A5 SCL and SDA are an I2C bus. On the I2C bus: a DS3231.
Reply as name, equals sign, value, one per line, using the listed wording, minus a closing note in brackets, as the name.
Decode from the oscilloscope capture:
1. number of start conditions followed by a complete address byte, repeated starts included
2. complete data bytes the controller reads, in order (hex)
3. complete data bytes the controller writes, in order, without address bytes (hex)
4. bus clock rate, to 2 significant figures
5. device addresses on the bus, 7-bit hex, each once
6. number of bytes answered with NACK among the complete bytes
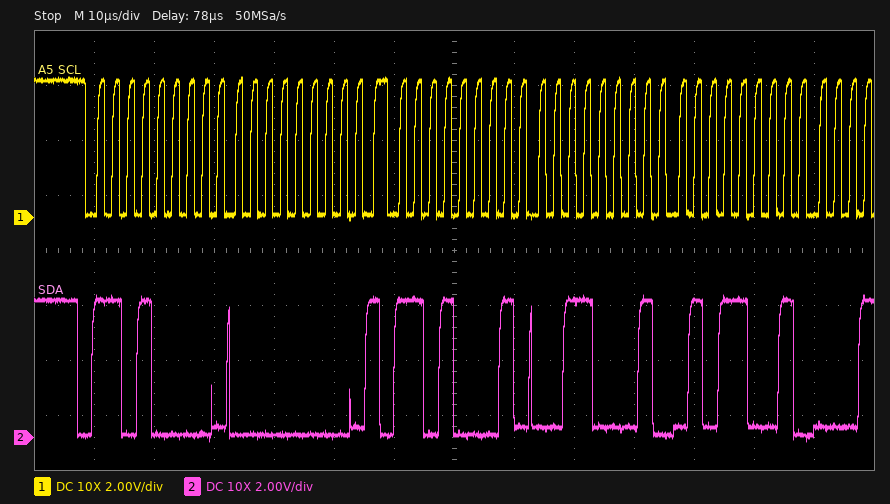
number of start conditions followed by a complete address byte, repeated starts included = 2
complete data bytes the controller reads, in order = 31 59
complete data bytes the controller writes, in order, without address bytes = 00
bus clock rate, to 2 significant figures = 400 kHz
device addresses on the bus, 7-bit hex, each once = 0x68
number of bytes answered with NACK among the complete bytes = 0
